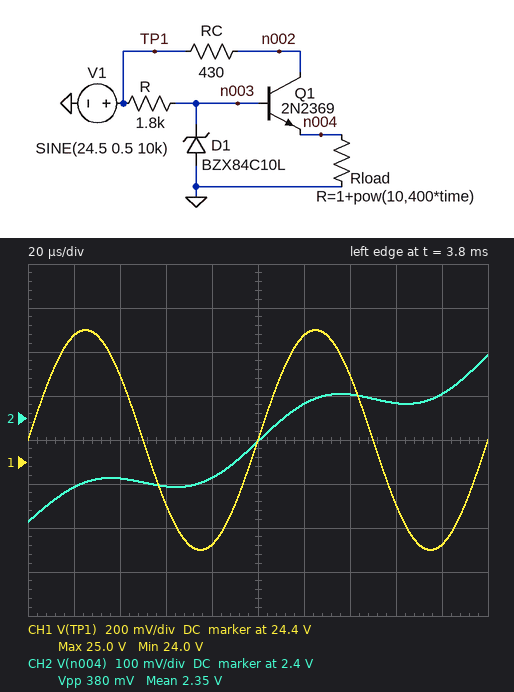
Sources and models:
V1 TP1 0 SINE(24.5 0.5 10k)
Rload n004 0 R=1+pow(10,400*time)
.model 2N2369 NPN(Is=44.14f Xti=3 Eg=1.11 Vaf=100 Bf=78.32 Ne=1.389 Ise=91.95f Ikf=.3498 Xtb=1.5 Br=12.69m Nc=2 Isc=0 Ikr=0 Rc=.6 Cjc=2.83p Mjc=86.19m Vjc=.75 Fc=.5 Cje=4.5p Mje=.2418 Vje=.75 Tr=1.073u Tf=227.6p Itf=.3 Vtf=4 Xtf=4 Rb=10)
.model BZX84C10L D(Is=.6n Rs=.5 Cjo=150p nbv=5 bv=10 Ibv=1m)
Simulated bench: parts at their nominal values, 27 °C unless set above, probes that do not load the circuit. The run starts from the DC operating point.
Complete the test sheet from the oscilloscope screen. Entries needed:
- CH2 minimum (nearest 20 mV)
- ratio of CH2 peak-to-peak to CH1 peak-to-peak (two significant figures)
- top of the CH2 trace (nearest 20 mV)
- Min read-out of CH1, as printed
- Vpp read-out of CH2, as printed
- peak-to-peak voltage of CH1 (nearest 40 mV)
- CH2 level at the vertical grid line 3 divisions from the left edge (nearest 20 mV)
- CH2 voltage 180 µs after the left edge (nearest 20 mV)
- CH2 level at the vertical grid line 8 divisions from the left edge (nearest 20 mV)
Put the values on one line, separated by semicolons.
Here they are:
2.16 V; 0.38; 2.54 V; 24.0 V; 380 mV; 1.00 V; 2.24 V; 2.46 V; 2.44 V
